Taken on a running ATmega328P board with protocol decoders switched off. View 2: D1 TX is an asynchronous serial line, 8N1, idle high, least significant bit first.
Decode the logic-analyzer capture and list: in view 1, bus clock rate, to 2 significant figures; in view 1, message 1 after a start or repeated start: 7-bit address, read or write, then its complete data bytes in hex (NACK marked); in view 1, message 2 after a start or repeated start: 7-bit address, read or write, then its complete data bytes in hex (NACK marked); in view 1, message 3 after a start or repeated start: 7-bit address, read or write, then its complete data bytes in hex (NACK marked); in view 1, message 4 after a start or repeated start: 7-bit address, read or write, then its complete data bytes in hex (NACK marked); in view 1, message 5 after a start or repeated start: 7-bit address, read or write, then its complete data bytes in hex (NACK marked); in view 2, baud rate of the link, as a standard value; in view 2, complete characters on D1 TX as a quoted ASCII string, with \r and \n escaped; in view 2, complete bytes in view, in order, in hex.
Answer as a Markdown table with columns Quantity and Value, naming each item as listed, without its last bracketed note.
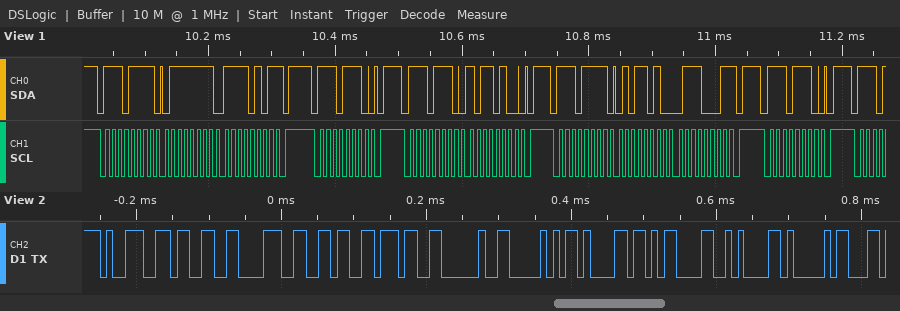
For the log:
| Quantity | Value |
|---|---|
| in view 1, bus clock rate, to 2 significant figures | 100 kHz |
| in view 1, message 1 after a start or repeated start: 7-bit address, read or write, then its complete data bytes in hex | 0x77 read: 7F F5 NACK |
| in view 1, message 2 after a start or repeated start: 7-bit address, read or write, then its complete data bytes in hex | 0x77 write |
| in view 1, message 3 after a start or repeated start: 7-bit address, read or write, then its complete data bytes in hex | 0x77 write: B4 |
| in view 1, message 4 after a start or repeated start: 7-bit address, read or write, then its complete data bytes in hex | 0x77 read: 5A 71 NACK |
| in view 1, message 5 after a start or repeated start: 7-bit address, read or write, then its complete data bytes in hex | 0x77 write |
| in view 2, baud rate of the link, as a standard value | 115200 baud |
| in view 2, complete characters on D1 TX as a quoted ASCII string, with \r and \n escaped | "93867 Pa\r\nA" |
| in view 2, complete bytes in view, in order, in hex | 39 33 38 36 37 20 50 61 0D 0A 41 |
